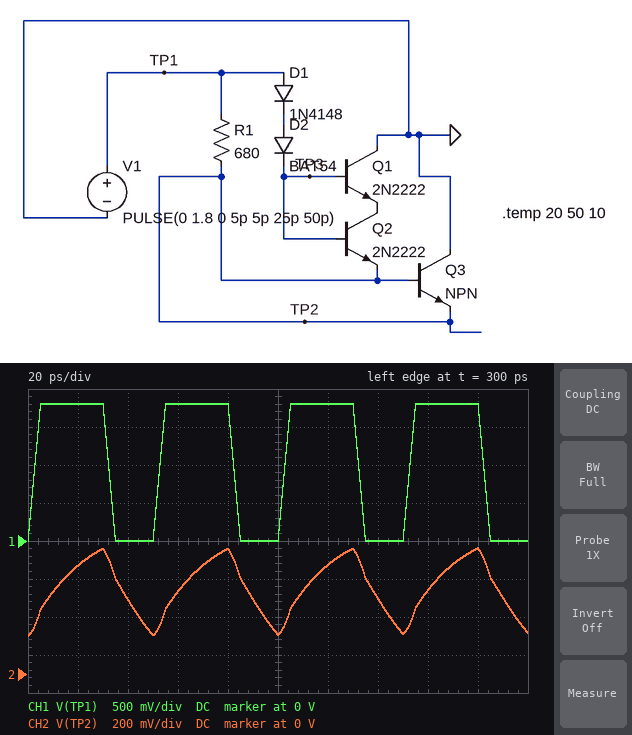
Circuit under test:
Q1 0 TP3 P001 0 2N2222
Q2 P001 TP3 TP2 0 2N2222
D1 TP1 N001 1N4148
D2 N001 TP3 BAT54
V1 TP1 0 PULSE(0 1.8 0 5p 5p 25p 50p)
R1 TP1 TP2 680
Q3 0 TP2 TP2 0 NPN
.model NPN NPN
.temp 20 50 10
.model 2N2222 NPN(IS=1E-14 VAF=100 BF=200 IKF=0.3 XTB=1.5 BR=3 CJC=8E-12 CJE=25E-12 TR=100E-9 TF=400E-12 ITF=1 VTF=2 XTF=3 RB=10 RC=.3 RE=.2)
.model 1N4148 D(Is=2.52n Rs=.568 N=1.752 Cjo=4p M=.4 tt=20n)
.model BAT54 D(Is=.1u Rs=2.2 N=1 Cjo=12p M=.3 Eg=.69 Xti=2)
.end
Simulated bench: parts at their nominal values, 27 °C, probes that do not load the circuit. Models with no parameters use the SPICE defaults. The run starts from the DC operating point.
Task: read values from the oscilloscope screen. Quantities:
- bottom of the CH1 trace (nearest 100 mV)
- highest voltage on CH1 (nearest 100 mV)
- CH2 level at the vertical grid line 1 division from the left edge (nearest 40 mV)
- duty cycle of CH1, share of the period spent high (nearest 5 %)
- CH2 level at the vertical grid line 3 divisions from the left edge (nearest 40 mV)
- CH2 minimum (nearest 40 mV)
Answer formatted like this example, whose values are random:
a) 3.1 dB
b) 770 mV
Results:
a) 0 V
b) 1.8 V
c) 560 mV
d) 60 %
e) 440 mV
f) 200 mV
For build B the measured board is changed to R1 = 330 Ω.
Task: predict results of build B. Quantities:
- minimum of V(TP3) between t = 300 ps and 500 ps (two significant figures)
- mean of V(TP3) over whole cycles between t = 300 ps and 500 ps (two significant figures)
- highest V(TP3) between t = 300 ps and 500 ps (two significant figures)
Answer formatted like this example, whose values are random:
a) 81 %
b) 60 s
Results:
a) -310 mV
b) 440 mV
c) 960 mV
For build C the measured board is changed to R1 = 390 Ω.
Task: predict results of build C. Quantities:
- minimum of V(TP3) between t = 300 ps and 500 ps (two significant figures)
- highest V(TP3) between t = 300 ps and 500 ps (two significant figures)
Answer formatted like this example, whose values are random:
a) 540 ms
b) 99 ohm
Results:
a) -310 mV
b) 950 mV
